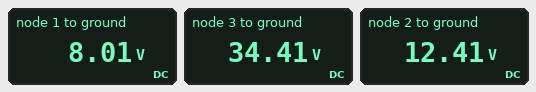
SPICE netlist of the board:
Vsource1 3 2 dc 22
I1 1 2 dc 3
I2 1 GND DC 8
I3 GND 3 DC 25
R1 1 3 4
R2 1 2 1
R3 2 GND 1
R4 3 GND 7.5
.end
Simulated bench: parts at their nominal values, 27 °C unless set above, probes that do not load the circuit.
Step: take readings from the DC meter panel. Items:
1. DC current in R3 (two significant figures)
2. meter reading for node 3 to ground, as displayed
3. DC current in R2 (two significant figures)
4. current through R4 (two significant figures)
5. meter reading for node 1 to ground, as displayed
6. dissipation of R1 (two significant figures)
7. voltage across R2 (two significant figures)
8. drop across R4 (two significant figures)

12 A
34.41 V
4.4 A
4.6 A
8.01 V
170 W
4.4 V
34 V
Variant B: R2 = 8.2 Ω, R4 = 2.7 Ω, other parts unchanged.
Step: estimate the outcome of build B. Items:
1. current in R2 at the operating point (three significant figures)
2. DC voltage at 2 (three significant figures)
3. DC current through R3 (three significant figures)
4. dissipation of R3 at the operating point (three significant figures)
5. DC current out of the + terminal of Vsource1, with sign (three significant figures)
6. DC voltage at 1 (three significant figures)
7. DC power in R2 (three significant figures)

1.80 A
6.46 V
6.46 A
41.7 W
-5.26 A
-8.33 V
26.7 W
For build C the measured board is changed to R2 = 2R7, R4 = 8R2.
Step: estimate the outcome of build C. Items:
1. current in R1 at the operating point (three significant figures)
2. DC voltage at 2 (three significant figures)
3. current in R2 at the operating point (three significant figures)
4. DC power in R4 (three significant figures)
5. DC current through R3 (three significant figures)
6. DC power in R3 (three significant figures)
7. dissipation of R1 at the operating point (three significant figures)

7.72 A
12.8 V
3.28 A
147 W
12.8 A
163 W
238 W
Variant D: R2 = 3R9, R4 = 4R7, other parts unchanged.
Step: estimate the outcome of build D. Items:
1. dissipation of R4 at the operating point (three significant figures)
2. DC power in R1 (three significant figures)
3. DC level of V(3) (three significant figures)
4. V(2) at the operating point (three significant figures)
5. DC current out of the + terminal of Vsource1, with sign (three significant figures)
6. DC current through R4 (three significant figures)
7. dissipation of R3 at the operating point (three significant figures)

220 W
270 W
32.2 V
10.2 V
-9.94 A
6.84 A
103 W
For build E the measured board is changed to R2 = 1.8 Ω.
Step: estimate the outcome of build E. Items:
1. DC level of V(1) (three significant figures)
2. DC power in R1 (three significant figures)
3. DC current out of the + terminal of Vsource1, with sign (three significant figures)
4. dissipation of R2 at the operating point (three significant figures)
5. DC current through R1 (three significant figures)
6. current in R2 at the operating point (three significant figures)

5.58 V
208 W
-13.2 A
25.9 W
7.21 A
3.79 A
